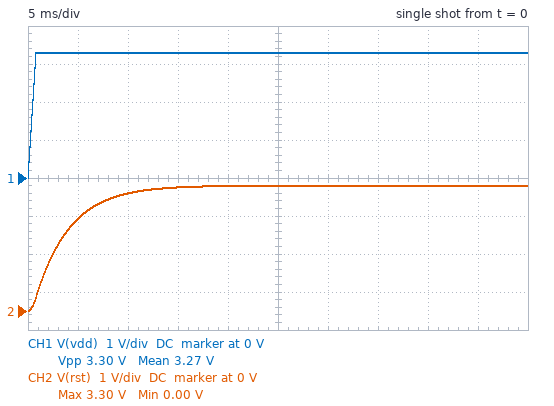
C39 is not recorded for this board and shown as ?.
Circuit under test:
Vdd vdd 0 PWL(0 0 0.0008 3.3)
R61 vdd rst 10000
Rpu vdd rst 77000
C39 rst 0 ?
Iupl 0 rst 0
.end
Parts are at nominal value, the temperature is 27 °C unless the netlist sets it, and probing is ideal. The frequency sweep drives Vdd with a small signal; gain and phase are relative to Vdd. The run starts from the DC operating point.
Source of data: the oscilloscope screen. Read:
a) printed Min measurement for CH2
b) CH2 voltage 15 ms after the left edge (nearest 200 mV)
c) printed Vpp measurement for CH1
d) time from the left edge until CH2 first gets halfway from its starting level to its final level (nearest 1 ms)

0.00 V
3.2 V
3.30 V
3 ms
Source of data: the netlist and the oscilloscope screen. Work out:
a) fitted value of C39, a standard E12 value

390 nF
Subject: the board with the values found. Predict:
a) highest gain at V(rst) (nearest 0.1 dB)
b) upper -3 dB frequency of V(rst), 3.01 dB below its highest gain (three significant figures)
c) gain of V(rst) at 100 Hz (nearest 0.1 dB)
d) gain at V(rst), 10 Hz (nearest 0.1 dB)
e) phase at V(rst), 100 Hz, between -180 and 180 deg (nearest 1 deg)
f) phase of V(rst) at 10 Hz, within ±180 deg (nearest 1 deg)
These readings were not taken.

0 dB
46.1 Hz
-7.6 dB
-0.2 dB
-65 deg
-12 deg
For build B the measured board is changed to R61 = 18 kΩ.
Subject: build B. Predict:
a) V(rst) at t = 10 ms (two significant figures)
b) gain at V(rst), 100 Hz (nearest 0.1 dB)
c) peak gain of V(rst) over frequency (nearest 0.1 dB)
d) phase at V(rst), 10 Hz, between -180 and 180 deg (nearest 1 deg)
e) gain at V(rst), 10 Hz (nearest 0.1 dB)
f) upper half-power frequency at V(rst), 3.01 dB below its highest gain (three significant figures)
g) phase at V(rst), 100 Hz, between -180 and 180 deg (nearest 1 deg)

2.7 V
-11.4 dB
0 dB
-20 deg
-0.5 dB
28.0 Hz
-74 deg
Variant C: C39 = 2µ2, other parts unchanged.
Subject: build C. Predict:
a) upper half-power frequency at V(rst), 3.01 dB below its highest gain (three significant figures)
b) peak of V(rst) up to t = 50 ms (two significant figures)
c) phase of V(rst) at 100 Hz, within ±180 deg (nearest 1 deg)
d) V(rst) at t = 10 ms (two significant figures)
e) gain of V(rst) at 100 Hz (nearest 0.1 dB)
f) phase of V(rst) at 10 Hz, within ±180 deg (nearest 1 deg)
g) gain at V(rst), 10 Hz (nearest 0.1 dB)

8.17 Hz
3.0 V
-85 deg
1.3 V
-21.8 dB
-51 deg
-4.0 dB
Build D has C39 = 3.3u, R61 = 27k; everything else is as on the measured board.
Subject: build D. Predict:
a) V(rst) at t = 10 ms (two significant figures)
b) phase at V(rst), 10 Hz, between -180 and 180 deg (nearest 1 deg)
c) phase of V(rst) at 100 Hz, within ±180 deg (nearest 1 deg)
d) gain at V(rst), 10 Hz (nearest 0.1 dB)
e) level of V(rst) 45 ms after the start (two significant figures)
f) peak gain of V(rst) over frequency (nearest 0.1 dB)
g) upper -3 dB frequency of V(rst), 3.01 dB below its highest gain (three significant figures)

450 mV
-76 deg
-89 deg
-12.6 dB
1.6 V
0 dB
2.41 Hz
